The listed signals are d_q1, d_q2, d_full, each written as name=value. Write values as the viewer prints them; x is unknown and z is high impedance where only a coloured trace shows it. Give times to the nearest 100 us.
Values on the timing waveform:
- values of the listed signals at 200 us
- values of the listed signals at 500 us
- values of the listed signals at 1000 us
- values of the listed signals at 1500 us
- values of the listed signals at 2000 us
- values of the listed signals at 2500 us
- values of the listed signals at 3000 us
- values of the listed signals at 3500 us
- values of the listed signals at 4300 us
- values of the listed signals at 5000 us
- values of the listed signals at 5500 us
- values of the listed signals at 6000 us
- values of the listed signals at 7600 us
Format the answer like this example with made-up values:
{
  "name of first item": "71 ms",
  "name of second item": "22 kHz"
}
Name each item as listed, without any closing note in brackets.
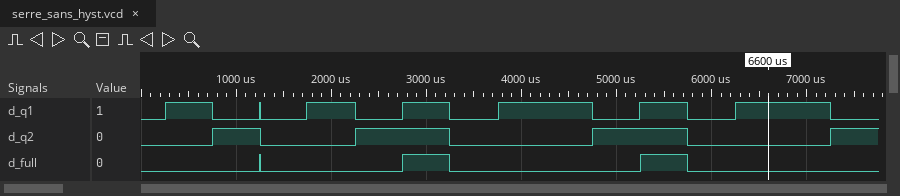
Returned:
{
  "values of the listed signals at 200 us": "d_q1=0, d_q2=0, d_full=0",
  "values of the listed signals at 500 us": "d_q1=1, d_q2=0, d_full=0",
  "values of the listed signals at 1000 us": "d_q1=0, d_q2=1, d_full=0",
  "values of the listed signals at 1500 us": "d_q1=0, d_q2=0, d_full=0",
  "values of the listed signals at 2000 us": "d_q1=1, d_q2=0, d_full=0",
  "values of the listed signals at 2500 us": "d_q1=0, d_q2=1, d_full=0",
  "values of the listed signals at 3000 us": "d_q1=1, d_q2=1, d_full=1",
  "values of the listed signals at 3500 us": "d_q1=0, d_q2=0, d_full=0",
  "values of the listed signals at 4300 us": "d_q1=1, d_q2=0, d_full=0",
  "values of the listed signals at 5000 us": "d_q1=0, d_q2=1, d_full=0",
  "values of the listed signals at 5500 us": "d_q1=1, d_q2=1, d_full=1",
  "values of the listed signals at 6000 us": "d_q1=0, d_q2=0, d_full=0",
  "values of the listed signals at 7600 us": "d_q1=0, d_q2=1, d_full=0"
}
